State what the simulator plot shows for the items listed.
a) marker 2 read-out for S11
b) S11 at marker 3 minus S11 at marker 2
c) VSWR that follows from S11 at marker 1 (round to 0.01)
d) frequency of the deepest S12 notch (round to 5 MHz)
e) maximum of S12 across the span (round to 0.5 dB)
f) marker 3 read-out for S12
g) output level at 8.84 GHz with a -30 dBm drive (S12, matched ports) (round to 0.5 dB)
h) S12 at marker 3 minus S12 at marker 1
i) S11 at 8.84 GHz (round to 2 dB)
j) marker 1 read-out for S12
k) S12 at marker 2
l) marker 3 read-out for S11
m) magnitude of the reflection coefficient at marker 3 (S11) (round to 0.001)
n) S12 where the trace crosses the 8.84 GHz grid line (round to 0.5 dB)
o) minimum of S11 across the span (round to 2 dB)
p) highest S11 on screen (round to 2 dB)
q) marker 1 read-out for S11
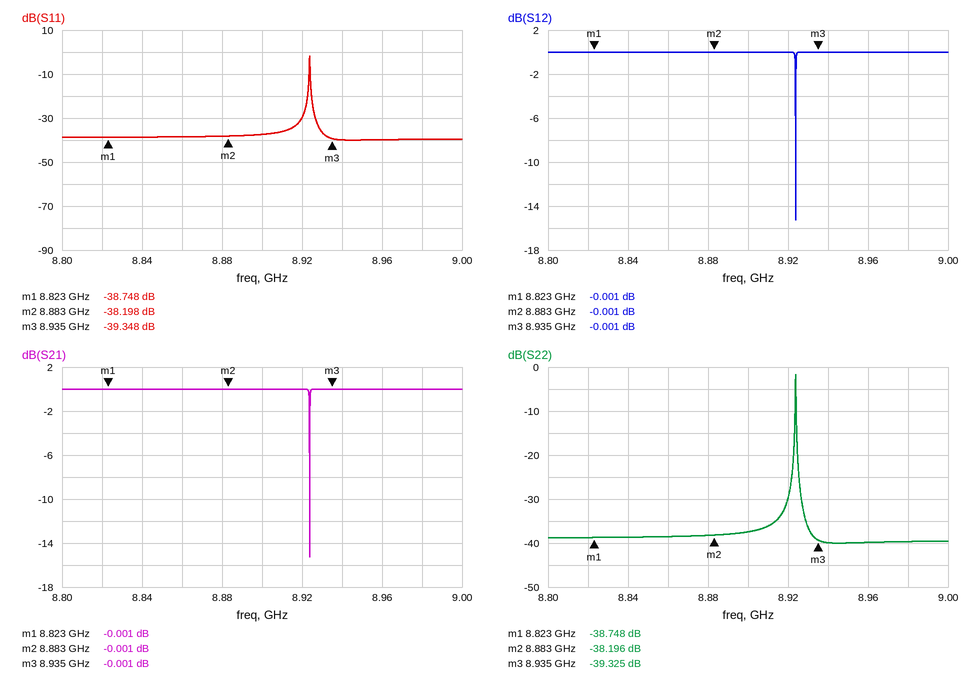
-38.198 dB
-1.150 dB
1.02
8.925 GHz
0.0 dB
-0.001 dB
-30.0 dBm
0.000 dB
-38 dB
-0.001 dB
-0.001 dB
-39.348 dB
0.011
0.0 dB
-40 dB
-2 dB
-38.748 dB
